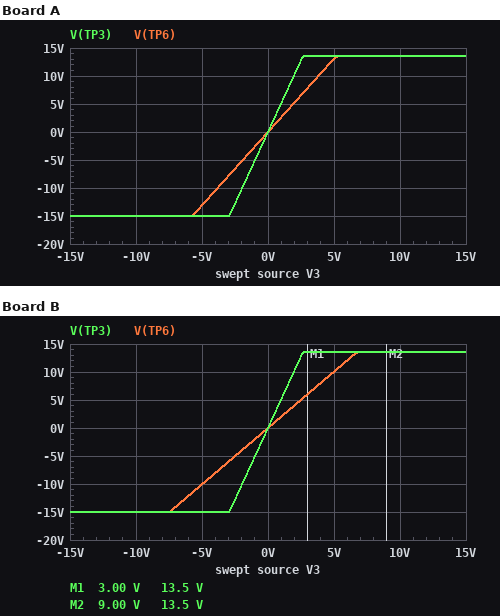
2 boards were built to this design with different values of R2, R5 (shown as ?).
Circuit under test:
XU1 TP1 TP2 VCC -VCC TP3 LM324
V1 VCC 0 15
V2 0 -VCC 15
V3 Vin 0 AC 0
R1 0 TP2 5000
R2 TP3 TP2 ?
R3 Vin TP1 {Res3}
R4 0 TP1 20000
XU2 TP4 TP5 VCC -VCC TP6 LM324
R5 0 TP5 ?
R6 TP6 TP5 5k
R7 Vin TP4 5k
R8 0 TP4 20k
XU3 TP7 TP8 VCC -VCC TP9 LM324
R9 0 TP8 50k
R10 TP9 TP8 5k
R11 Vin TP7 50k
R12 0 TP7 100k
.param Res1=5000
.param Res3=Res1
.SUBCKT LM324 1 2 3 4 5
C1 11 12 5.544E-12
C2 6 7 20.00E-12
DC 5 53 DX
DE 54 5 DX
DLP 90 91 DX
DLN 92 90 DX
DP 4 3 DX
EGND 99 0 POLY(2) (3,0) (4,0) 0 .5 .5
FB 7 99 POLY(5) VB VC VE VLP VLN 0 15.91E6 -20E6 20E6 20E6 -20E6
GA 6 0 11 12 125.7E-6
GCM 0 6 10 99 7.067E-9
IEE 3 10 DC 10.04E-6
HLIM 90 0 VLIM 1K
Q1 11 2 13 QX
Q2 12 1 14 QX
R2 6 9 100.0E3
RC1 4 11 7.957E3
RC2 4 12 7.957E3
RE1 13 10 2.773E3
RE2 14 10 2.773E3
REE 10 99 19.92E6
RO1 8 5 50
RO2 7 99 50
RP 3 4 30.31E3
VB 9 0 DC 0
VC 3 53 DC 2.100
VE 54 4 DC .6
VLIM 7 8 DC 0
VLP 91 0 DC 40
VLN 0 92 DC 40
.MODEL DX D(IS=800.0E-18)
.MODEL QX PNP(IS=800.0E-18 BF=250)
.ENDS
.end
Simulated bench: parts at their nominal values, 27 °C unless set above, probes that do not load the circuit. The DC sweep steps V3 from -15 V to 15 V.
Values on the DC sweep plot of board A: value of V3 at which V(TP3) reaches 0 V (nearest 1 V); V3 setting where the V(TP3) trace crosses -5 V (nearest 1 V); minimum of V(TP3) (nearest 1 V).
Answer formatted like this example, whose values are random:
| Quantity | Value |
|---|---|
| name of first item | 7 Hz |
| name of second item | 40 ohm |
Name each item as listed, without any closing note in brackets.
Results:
| Quantity | Value |
|---|---|
| value of V3 at which V(TP3) reaches 0 V | 0 V |
| V3 setting where the V(TP3) trace crosses -5 V | -1 V |
| minimum of V(TP3) | -15 V |
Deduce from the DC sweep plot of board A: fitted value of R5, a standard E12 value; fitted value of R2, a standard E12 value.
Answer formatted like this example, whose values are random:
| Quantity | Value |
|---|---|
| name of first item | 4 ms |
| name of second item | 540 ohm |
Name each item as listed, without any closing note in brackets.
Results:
| Quantity | Value |
|---|---|
| fitted value of R5, a standard E12 value | 2.2 kΩ |
| fitted value of R2, a standard E12 value | 27 kΩ |
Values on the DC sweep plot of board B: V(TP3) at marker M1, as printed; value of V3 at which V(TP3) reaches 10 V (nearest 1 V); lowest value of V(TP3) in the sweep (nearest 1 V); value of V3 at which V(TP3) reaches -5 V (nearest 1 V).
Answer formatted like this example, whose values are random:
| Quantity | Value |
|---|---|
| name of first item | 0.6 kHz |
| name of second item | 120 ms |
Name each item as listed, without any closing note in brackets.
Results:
| Quantity | Value |
|---|---|
| V(TP3) at marker M1, as printed | 13.5 V |
| value of V3 at which V(TP3) reaches 10 V | 2 V |
| lowest value of V(TP3) in the sweep | -15 V |
| value of V3 at which V(TP3) reaches -5 V | -1 V |
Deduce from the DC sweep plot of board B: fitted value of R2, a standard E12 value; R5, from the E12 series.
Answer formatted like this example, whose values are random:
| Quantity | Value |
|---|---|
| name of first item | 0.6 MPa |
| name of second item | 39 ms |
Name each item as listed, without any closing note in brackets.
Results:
| Quantity | Value |
|---|---|
| fitted value of R2, a standard E12 value | 27 kΩ |
| R5, from the E12 series | 3.3 kΩ |
